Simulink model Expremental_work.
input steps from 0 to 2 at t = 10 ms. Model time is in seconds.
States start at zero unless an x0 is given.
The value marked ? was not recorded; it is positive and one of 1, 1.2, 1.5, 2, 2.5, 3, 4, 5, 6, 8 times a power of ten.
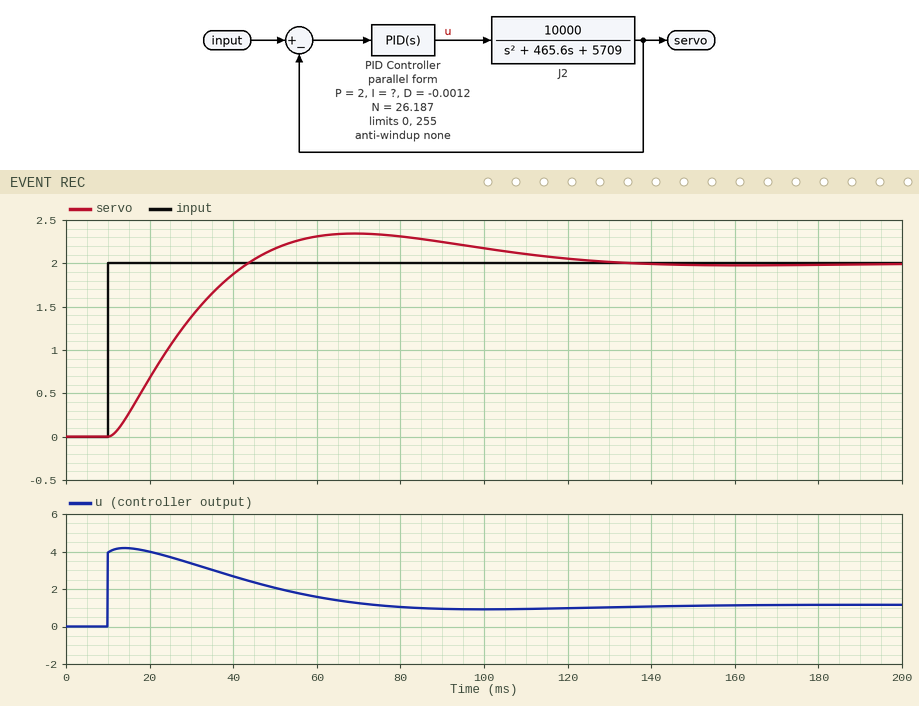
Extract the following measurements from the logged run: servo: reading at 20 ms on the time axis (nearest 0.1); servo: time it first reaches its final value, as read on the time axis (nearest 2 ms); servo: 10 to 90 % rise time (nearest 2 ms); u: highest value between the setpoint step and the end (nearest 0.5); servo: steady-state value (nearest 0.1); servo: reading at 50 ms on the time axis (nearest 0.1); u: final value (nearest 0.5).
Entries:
0.7
44 ms
24 ms
4.0
2.0
2.2
1.0
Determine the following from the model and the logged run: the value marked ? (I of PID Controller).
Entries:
80
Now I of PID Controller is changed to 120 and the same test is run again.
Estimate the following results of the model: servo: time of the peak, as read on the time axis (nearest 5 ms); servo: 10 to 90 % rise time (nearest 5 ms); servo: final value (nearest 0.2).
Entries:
60 ms
20 ms
2.0
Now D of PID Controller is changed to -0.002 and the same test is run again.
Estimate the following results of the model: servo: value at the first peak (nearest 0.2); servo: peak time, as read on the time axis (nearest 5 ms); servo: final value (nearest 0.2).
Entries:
2.4
70 ms
2.0
